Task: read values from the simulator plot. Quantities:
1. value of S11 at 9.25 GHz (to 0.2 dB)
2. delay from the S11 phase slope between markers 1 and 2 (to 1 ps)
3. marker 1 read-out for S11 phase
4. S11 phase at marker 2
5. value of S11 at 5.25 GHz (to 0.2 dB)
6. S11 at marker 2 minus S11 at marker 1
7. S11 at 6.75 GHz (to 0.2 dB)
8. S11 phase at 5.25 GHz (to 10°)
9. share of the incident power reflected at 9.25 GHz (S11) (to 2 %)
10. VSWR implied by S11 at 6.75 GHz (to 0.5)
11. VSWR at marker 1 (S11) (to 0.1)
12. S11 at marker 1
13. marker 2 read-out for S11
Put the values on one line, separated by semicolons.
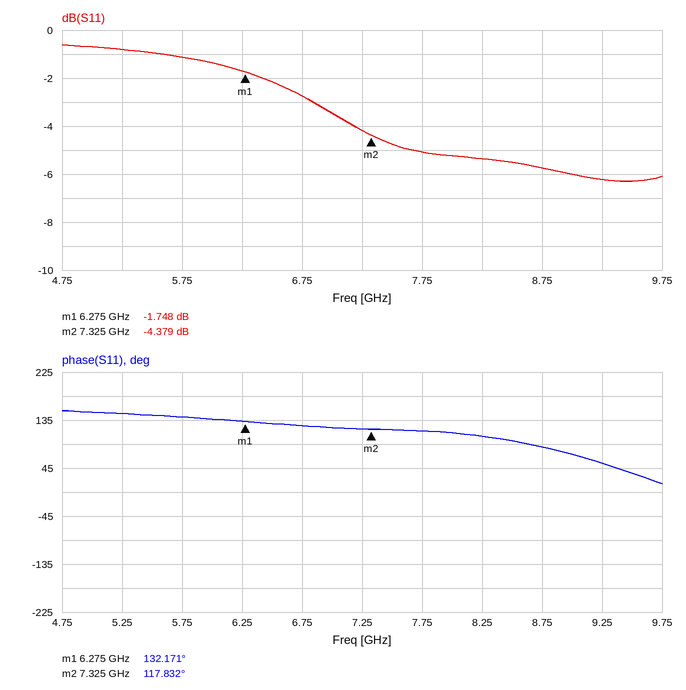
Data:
-6.2 dB; 38 ps; 132.171°; 117.832°; -0.8 dB; -2.631 dB; -2.8 dB; 150°; 24 %; 6.5; 10.0; -1.748 dB; -4.379 dB
